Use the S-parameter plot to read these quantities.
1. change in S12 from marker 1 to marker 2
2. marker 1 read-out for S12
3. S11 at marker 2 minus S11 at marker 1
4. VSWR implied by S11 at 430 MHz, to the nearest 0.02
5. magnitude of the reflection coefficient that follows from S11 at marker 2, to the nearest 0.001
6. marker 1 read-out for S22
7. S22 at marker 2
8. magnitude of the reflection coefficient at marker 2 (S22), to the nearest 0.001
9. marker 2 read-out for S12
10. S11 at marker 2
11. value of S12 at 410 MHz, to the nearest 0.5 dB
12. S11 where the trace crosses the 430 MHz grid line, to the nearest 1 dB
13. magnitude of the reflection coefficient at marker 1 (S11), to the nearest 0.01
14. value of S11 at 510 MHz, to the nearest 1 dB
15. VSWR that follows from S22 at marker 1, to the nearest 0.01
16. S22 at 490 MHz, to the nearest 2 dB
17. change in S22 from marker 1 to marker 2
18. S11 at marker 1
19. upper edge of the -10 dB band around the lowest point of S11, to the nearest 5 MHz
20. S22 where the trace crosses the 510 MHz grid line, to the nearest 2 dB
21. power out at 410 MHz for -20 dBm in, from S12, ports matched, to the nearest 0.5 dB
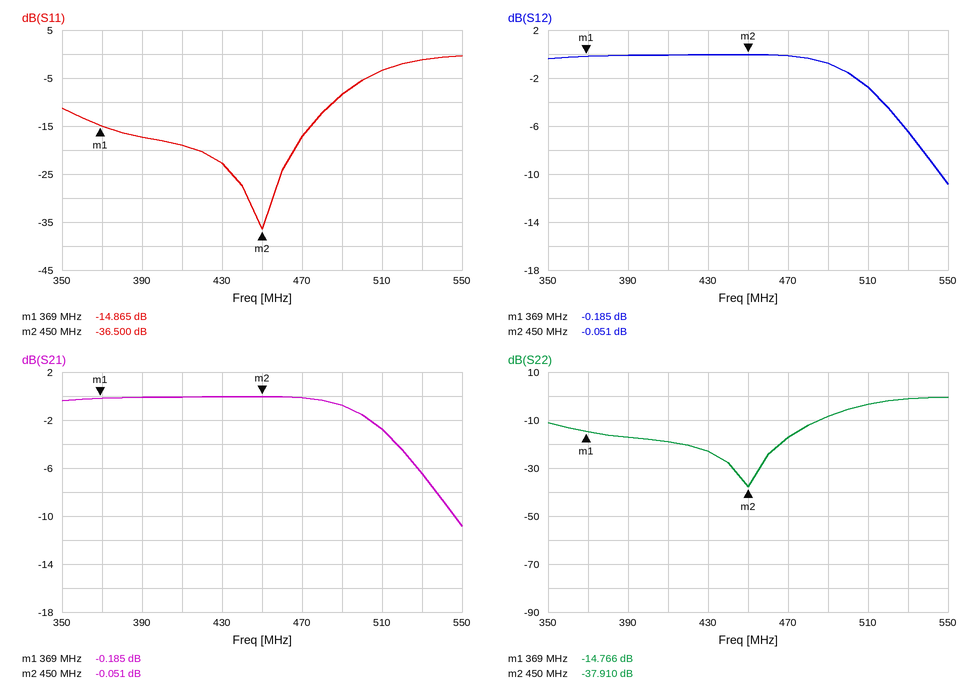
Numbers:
0.134 dB
-0.185 dB
-21.635 dB
1.16
0.015
-14.766 dB
-37.910 dB
0.013
-0.051 dB
-36.500 dB
0.0 dB
-23 dB
0.18
-3 dB
1.45
-8 dB
-23.144 dB
-14.865 dB
485 MHz
-4 dB
-20.0 dBm
